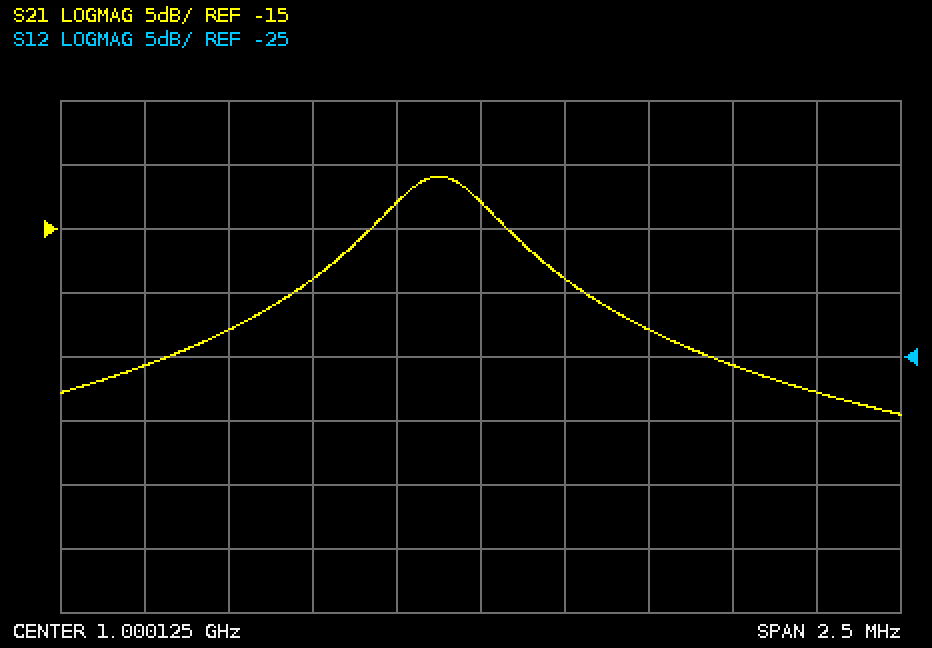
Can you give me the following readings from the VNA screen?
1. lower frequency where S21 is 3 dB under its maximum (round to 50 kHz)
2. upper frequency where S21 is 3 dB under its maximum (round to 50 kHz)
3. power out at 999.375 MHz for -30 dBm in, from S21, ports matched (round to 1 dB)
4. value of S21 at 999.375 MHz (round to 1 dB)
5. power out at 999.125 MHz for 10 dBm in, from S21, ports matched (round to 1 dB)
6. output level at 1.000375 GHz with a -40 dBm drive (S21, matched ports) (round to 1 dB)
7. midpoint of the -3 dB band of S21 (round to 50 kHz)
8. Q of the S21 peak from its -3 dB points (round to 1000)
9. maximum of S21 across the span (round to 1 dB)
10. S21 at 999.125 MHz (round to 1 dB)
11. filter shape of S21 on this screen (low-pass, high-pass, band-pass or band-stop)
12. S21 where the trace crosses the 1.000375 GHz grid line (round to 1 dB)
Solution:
999.85 MHz
1.00015 GHz
-53 dBm
-23 dB
-16 dBm
-59 dBm
1.00000 GHz
3000
-11 dB
-26 dB
band-pass
-19 dB
